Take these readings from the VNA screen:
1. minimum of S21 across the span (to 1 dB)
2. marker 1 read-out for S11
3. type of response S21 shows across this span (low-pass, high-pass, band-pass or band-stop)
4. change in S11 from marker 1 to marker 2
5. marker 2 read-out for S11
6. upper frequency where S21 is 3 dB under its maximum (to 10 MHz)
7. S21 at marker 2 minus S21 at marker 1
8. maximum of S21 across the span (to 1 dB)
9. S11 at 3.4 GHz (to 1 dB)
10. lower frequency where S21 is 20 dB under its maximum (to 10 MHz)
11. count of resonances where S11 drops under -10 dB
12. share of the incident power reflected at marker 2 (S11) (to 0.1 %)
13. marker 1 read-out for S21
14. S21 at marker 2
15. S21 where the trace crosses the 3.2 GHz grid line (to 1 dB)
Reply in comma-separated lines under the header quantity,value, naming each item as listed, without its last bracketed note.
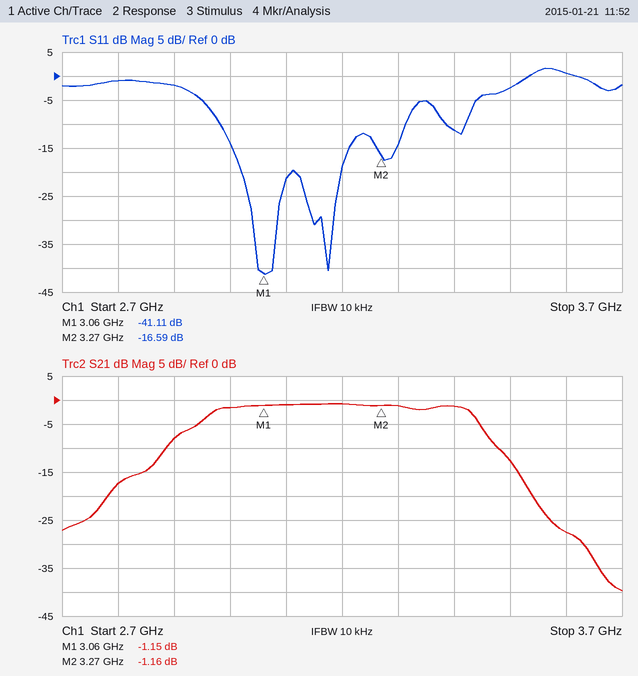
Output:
quantity,value
minimum of S21 across the span,-40 dB
marker 1 read-out for S11,-41.11 dB
type of response S21 shows across this span,band-pass
change in S11 from marker 1 to marker 2,24.52 dB
marker 2 read-out for S11,-16.59 dB
upper frequency where S21 is 3 dB under its maximum,3.44 GHz
S21 at marker 2 minus S21 at marker 1,-0.01 dB
maximum of S21 across the span,-1 dB
S11 at 3.4 GHz,-11 dB
lower frequency where S21 is 20 dB under its maximum,2.78 GHz
count of resonances where S11 drops under -10 dB,4
share of the incident power reflected at marker 2 (S11),2.2 %
marker 1 read-out for S21,-1.15 dB
S21 at marker 2,-1.16 dB
S21 where the trace crosses the 3.2 GHz grid line,-1 dB
